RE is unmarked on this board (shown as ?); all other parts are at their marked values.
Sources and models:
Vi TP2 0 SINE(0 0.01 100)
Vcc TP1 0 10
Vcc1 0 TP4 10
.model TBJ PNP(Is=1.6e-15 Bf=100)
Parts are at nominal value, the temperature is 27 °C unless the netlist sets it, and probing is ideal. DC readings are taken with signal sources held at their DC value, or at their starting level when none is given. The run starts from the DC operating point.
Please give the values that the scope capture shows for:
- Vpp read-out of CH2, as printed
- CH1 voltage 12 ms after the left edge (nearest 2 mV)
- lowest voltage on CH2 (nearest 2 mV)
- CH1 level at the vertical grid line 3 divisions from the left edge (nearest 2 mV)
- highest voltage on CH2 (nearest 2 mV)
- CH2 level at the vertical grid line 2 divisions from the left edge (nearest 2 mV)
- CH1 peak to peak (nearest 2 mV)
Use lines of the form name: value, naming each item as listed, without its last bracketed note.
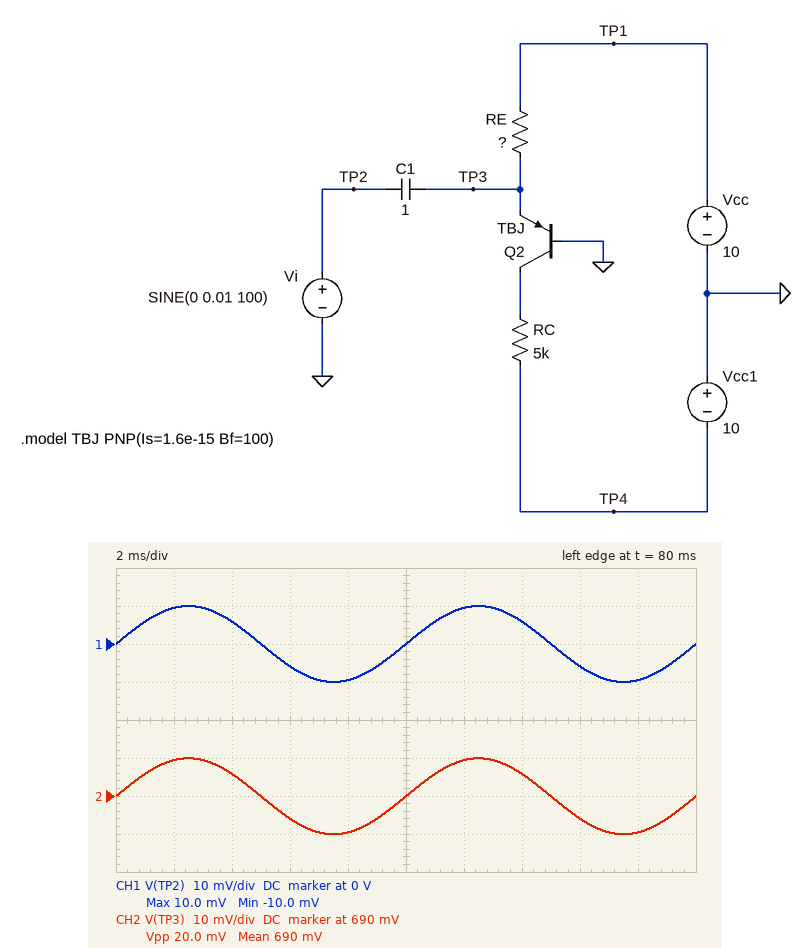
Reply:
Vpp read-out of CH2, as printed: 20.0 mV
CH1 voltage 12 ms after the left edge: 10 mV
lowest voltage on CH2: 680 mV
CH1 level at the vertical grid line 3 divisions from the left edge: -6 mV
highest voltage on CH2: 700 mV
CH2 level at the vertical grid line 2 divisions from the left edge: 696 mV
CH1 peak to peak: 20 mV
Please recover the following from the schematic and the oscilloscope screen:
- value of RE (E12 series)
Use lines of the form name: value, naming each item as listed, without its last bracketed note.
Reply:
value of RE: 15 kΩ
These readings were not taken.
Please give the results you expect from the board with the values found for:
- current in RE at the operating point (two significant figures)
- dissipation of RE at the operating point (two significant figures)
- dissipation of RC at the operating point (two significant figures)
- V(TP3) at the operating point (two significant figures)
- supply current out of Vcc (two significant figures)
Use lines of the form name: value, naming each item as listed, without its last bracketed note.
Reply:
current in RE at the operating point: 620 µA
dissipation of RE at the operating point: 5.8 mW
dissipation of RC at the operating point: 1.9 mW
V(TP3) at the operating point: 690 mV
supply current out of Vcc: 620 µA
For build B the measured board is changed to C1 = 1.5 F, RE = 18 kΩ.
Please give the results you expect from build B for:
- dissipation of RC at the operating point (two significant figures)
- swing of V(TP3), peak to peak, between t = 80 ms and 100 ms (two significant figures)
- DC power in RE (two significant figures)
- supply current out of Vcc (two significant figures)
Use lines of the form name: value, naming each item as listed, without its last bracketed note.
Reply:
dissipation of RC at the operating point: 1.3 mW
swing of V(TP3), peak to peak, between t = 80 ms and 100 ms: 20 mV
DC power in RE: 4.8 mW
supply current out of Vcc: 520 µA
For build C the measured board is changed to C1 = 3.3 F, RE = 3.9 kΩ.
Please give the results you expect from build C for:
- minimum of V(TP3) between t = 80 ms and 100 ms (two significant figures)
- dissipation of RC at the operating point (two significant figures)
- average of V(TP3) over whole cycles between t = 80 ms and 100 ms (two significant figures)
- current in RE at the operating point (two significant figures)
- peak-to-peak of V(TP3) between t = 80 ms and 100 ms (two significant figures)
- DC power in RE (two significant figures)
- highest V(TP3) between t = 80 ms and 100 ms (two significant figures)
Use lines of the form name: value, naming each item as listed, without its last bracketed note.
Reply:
minimum of V(TP3) between t = 80 ms and 100 ms: 720 mV
dissipation of RC at the operating point: 23 mW
average of V(TP3) over whole cycles between t = 80 ms and 100 ms: 730 mV
current in RE at the operating point: 2.4 mA
peak-to-peak of V(TP3) between t = 80 ms and 100 ms: 20 mV
DC power in RE: 22 mW
highest V(TP3) between t = 80 ms and 100 ms: 740 mV
